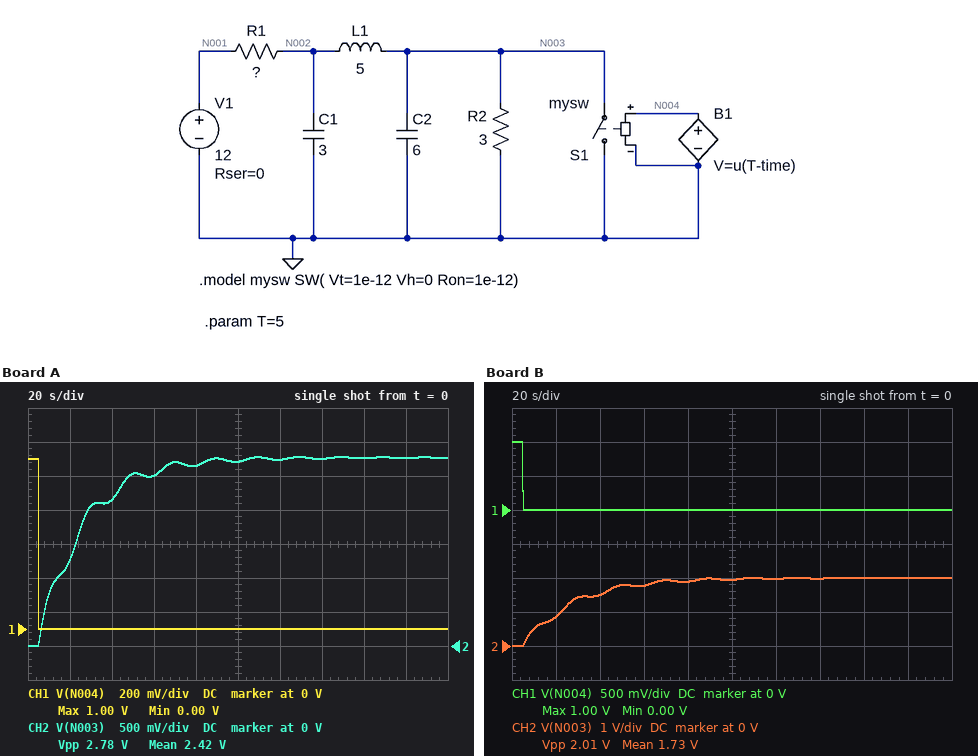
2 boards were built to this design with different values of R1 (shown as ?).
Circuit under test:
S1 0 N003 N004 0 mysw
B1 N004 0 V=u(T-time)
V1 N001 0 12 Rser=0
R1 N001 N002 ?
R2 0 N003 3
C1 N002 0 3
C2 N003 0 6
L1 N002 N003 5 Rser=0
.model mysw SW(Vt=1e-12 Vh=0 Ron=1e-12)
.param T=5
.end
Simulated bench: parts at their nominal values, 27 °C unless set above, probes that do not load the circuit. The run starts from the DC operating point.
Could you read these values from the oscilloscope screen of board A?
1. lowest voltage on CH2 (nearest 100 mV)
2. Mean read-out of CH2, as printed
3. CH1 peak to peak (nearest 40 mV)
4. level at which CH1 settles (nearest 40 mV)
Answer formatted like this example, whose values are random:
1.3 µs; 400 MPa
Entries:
0 V; 2.42 V; 1.00 V; 0 V
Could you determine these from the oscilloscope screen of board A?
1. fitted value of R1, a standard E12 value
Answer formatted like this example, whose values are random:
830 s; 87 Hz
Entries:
10 Ω
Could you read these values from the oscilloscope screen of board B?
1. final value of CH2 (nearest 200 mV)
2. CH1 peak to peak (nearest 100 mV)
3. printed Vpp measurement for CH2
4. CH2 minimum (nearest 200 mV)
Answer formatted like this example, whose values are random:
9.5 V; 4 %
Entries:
2.0 V; 1.0 V; 2.01 V; 0 V
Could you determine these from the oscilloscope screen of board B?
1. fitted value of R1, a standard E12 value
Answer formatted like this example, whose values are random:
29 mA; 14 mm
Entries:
15 Ω
